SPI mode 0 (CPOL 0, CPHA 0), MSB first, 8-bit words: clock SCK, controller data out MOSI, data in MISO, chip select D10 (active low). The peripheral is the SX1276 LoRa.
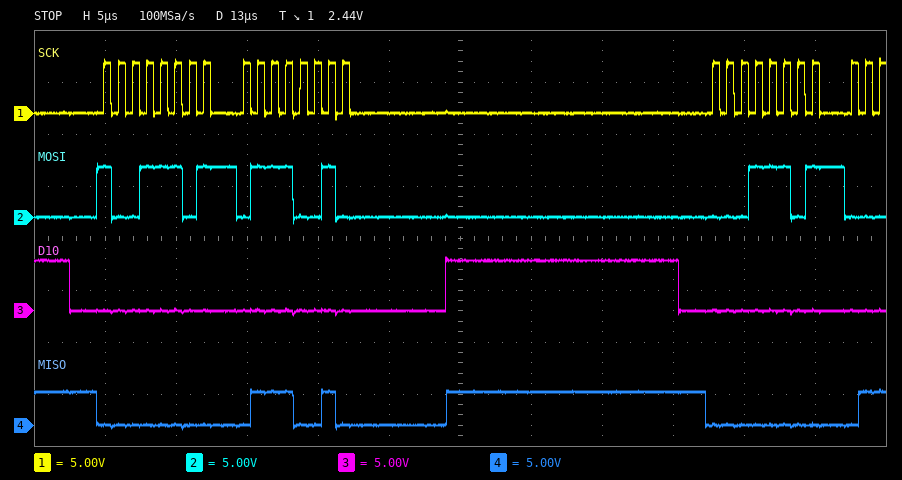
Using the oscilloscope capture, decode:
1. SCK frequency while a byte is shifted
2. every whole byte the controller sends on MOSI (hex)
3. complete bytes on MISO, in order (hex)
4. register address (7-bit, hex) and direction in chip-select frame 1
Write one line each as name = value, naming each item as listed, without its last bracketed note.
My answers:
SCK frequency while a byte is shifted = 1 MHz
every whole byte the controller sends on MOSI = 9D 72 1D
complete bytes on MISO, in order = 00 72 00
register address (7-bit, hex) and direction in chip-select frame 1 = 0x1D write
